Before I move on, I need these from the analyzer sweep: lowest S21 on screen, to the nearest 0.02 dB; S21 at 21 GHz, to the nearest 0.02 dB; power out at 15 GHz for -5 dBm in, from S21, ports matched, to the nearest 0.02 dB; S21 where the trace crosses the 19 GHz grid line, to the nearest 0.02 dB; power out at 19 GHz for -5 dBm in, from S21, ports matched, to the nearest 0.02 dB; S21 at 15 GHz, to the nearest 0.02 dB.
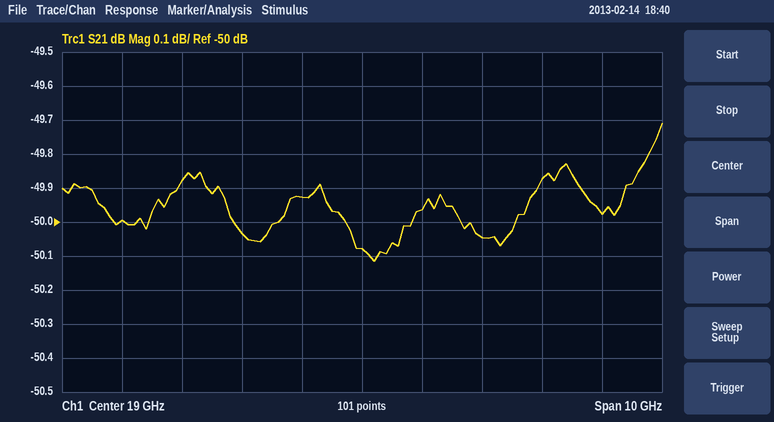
-50.12 dB
-50.04 dB
-55.00 dBm
-50.08 dB
-55.08 dBm
-50.00 dB
